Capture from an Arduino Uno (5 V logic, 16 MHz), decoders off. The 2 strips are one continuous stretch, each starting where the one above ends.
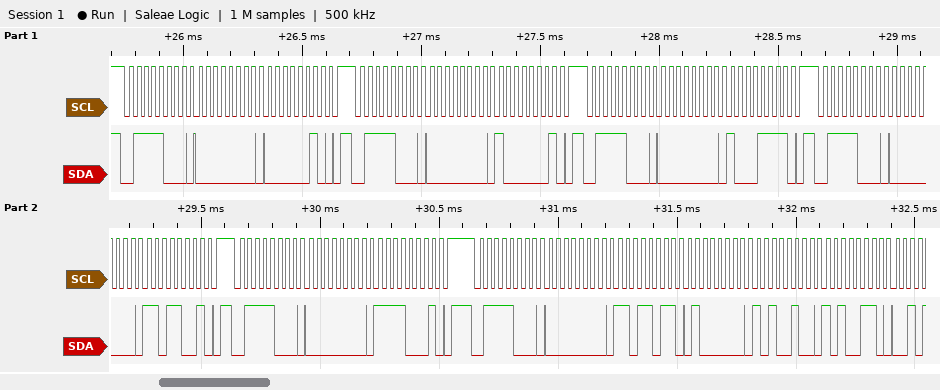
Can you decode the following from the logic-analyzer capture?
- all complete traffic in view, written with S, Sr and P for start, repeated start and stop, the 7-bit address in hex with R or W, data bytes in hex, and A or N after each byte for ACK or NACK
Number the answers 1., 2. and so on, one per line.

1. S 3CW A 00 A 02 A P S 3CW A 00 A 81 A P S 3CW A 00 A 8F A P S 3CW A 00 A D9 A P S 3CW A 00 A F1 A P S 3CW A 00 A DB A 40 A A4 A A6 A
